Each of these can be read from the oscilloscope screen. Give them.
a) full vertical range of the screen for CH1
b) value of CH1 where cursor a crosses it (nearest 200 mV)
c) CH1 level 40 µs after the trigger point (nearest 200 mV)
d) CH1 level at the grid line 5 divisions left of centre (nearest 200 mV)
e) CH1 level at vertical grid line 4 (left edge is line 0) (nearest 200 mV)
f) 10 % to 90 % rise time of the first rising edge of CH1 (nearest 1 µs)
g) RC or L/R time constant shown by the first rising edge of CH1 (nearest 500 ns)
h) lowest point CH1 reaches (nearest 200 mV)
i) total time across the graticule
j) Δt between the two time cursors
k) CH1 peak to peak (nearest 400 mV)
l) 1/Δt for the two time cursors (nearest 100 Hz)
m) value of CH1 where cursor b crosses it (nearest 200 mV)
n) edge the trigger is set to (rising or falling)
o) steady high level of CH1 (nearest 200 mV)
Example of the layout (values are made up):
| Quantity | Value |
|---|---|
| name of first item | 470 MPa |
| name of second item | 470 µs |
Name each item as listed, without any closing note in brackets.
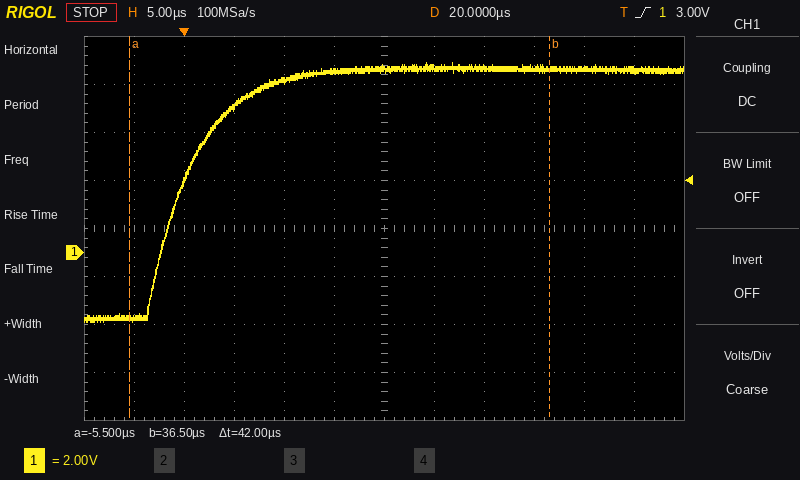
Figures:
| Quantity | Value |
|---|---|
| full vertical range of the screen for CH1 | 16 V |
| value of CH1 where cursor a crosses it | -2.8 V |
| CH1 level 40 µs after the trigger point | 7.6 V |
| CH1 level at the grid line 5 divisions left of centre | -2.8 V |
| CH1 level at vertical grid line 4 (left edge is line 0) | 7.2 V |
| 10 % to 90 % rise time of the first rising edge of CH1 | 10 µs |
| RC or L/R time constant shown by the first rising edge of CH1 | 4.5 µs |
| lowest point CH1 reaches | -2.8 V |
| total time across the graticule | 60 µs |
| Δt between the two time cursors | 42 µs |
| CH1 peak to peak | 10.8 V |
| 1/Δt for the two time cursors | 23.8 kHz |
| value of CH1 where cursor b crosses it | 7.6 V |
| edge the trigger is set to | rising |
| steady high level of CH1 | 7.6 V |
